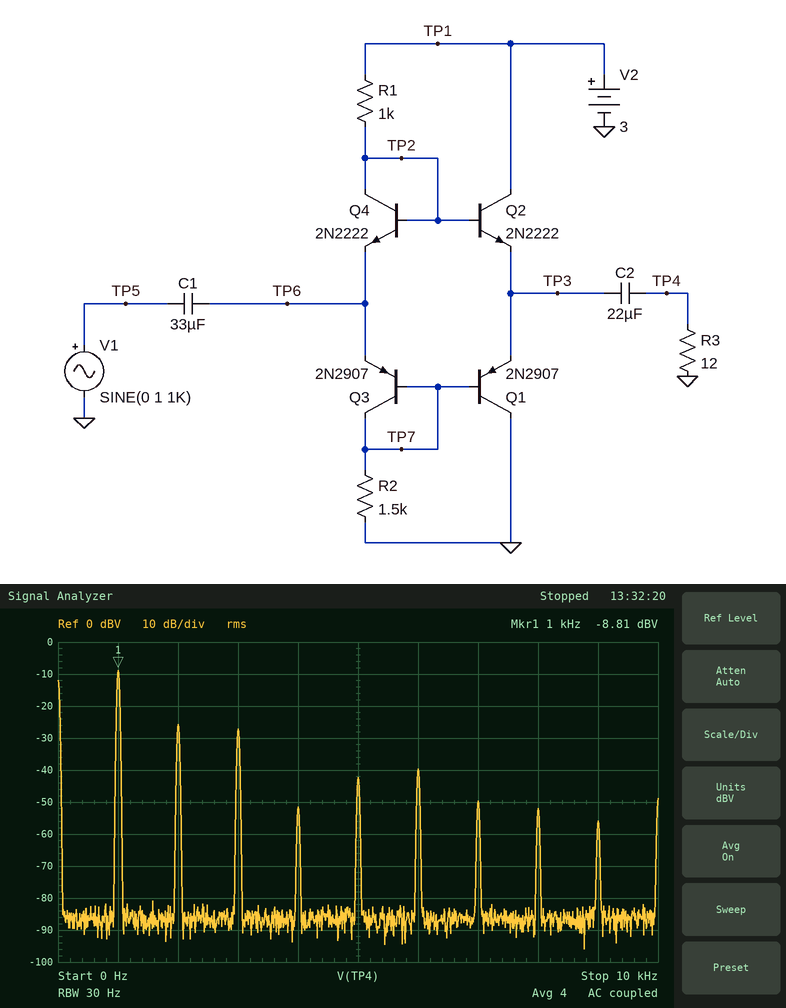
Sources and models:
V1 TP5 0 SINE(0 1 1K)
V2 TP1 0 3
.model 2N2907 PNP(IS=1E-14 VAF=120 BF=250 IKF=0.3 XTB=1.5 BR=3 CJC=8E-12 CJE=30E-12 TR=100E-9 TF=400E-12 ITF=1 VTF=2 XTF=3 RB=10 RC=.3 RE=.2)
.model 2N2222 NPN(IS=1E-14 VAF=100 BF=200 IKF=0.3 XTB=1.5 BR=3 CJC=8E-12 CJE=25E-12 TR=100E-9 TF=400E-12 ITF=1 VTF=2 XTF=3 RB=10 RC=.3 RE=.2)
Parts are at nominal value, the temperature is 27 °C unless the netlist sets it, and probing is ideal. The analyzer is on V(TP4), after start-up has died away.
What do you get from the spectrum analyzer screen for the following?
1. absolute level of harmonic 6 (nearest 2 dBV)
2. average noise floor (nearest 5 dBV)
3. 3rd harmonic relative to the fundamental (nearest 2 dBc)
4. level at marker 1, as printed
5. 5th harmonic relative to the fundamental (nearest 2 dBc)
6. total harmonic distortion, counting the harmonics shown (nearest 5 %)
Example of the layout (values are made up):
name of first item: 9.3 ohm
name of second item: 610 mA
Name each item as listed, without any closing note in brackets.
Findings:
absolute level of harmonic 6: -40 dBV
average noise floor: -85 dBV
3rd harmonic relative to the fundamental: -18 dBc
level at marker 1, as printed: -8.81 dBV
5th harmonic relative to the fundamental: -34 dBc
total harmonic distortion, counting the harmonics shown: 20 %
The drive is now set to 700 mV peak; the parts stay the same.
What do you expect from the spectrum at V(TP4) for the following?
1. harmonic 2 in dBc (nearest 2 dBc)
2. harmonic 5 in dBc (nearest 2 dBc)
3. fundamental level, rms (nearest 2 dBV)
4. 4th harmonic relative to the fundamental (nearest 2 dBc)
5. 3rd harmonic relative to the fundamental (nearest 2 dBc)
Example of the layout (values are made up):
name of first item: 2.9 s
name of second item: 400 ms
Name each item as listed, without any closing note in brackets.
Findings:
harmonic 2 in dBc: -24 dBc
harmonic 5 in dBc: -32 dBc
fundamental level, rms: -10 dBV
4th harmonic relative to the fundamental: -32 dBc
3rd harmonic relative to the fundamental: -28 dBc
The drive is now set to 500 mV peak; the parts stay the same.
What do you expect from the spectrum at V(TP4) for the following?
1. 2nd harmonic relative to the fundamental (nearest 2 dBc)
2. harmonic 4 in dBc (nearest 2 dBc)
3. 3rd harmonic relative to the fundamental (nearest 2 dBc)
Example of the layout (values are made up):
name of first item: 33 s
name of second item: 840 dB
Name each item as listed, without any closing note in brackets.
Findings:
2nd harmonic relative to the fundamental: -38 dBc
harmonic 4 in dBc: -52 dBc
3rd harmonic relative to the fundamental: -26 dBc
